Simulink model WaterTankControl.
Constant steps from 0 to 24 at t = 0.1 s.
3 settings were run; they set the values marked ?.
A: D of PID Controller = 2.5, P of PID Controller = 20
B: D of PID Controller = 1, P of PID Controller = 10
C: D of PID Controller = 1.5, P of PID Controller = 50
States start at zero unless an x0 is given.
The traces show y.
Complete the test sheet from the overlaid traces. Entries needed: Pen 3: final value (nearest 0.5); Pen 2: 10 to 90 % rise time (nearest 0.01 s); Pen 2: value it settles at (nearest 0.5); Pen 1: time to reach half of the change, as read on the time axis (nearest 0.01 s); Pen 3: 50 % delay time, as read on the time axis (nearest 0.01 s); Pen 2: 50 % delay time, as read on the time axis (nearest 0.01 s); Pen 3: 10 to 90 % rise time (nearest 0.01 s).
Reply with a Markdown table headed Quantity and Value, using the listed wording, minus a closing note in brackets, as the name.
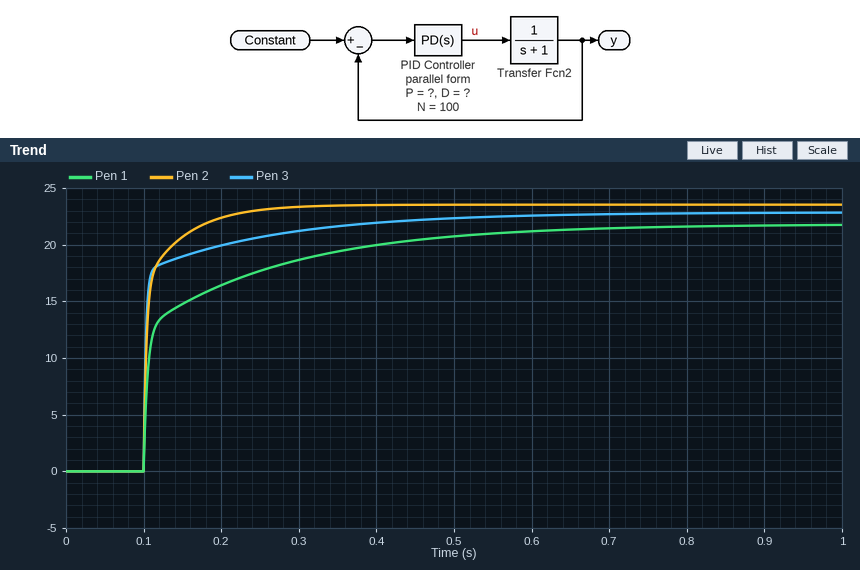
| Quantity | Value |
|---|---|
| Pen 3: final value | 23.0 |
| Pen 2: 10 to 90 % rise time | 0.06 s |
| Pen 2: value it settles at | 23.5 |
| Pen 1: time to reach half of the change, as read on the time axis | 0.11 s |
| Pen 3: 50 % delay time, as read on the time axis | 0.10 s |
| Pen 2: 50 % delay time, as read on the time axis | 0.10 s |
| Pen 3: 10 to 90 % rise time | 0.14 s |
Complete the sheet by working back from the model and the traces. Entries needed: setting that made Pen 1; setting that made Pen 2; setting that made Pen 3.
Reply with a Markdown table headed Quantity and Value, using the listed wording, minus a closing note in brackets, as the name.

| Quantity | Value |
|---|---|
| setting that made Pen 1 | B |
| setting that made Pen 2 | C |
| setting that made Pen 3 | A |
